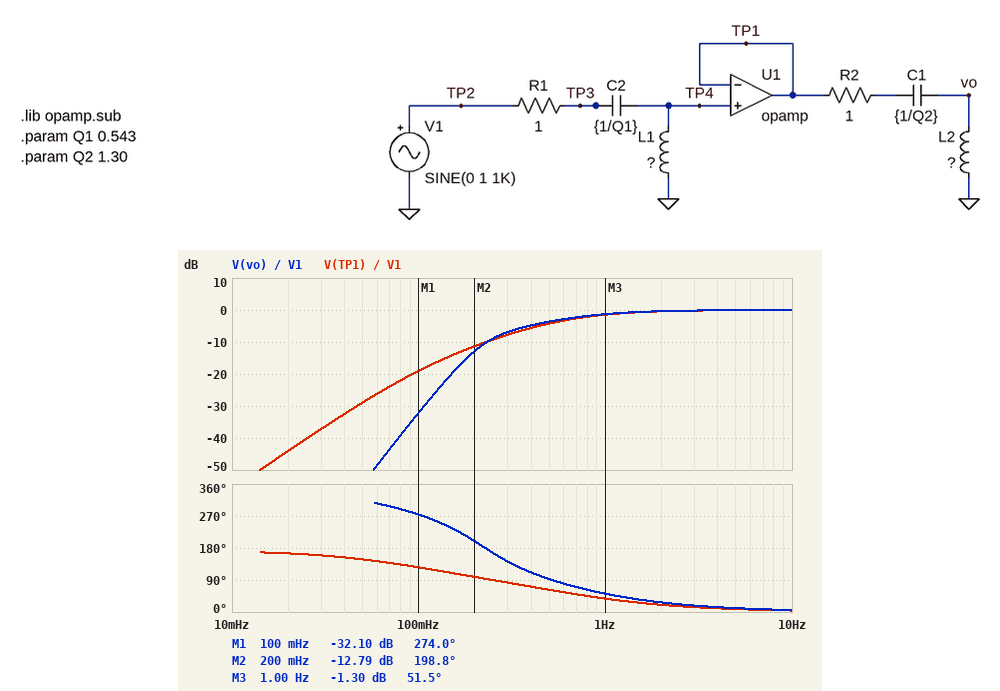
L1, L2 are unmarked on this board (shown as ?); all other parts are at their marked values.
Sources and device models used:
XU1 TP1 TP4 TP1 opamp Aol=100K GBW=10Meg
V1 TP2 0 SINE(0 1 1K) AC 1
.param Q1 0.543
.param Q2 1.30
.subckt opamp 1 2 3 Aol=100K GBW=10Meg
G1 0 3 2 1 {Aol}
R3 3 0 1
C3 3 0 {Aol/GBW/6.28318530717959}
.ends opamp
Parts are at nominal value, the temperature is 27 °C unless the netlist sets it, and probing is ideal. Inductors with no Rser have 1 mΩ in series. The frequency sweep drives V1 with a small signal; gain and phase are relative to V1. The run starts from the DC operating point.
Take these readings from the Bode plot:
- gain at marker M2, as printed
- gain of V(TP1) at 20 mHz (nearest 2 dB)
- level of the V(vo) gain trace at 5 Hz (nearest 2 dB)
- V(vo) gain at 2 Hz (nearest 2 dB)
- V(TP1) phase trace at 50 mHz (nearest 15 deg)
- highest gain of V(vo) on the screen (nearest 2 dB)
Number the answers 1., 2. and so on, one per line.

1. -12.79 dB
2. -44 dB
3. 0 dB
4. 0 dB
5. 150 deg
6. 0 dB
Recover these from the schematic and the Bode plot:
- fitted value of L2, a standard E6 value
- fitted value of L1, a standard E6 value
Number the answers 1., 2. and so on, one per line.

1. 680 mH
2. 220 mH
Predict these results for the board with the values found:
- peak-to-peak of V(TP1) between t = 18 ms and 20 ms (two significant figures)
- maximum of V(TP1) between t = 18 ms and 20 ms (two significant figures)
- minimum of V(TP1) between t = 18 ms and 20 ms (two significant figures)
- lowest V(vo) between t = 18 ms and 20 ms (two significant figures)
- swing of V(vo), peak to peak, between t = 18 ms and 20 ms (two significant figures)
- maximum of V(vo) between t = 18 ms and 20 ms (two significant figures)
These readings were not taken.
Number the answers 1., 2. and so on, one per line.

1. 2.0 V
2. 1.0 V
3. -1.0 V
4. -1.0 V
5. 2.0 V
6. 1.0 V
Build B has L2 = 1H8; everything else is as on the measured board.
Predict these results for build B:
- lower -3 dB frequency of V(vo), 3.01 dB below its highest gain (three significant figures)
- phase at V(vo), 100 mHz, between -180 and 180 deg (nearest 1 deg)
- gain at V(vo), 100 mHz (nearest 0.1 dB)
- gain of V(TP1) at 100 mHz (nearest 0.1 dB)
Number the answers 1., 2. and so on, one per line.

1. 592 mHz
2. -101 deg
3. -20.7 dB
4. -19.0 dB
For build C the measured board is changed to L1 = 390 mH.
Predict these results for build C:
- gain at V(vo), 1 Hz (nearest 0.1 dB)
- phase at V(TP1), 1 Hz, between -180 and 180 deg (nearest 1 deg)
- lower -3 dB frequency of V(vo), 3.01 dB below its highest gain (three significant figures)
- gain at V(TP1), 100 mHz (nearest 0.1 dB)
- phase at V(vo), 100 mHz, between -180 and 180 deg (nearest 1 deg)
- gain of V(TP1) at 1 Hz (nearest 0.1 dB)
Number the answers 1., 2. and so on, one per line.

1. -0.2 dB
2. 23 deg
3. 284 mHz
4. -13.6 dB
5. -90 deg
6. -0.4 dB
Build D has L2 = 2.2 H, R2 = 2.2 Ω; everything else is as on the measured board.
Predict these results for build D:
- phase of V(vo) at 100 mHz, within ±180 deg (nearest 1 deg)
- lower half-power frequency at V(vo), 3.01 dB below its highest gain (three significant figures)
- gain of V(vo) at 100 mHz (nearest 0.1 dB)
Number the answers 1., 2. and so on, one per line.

1. -127 deg
2. 633 mHz
3. -23.5 dB
